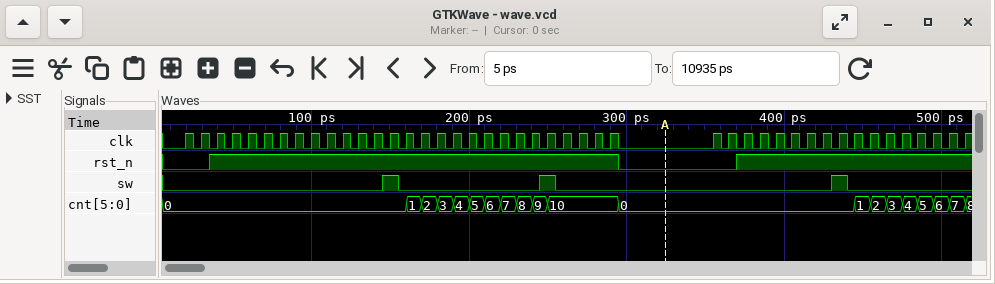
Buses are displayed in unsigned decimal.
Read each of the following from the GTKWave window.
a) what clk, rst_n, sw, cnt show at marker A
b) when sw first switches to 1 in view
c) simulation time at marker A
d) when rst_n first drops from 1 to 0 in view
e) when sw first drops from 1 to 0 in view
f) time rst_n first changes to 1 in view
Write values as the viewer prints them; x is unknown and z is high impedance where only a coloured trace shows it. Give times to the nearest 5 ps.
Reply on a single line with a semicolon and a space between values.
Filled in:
clk=0, rst_n=0, sw=0, cnt=0; 145 ps; 325 ps; 295 ps; 155 ps; 35 ps
